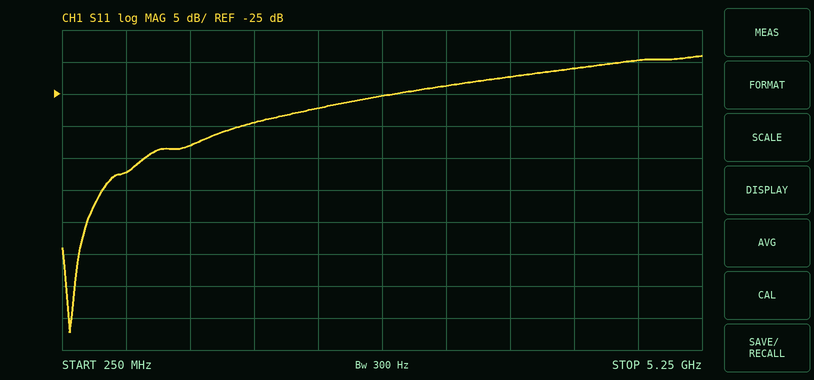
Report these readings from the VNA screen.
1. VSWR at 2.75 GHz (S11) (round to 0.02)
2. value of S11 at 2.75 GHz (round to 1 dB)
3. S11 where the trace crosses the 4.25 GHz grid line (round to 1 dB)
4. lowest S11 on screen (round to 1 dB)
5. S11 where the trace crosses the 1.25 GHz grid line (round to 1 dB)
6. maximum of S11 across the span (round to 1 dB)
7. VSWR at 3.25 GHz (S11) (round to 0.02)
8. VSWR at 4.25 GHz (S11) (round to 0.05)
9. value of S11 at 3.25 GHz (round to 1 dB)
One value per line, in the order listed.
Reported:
1.12
-25 dB
-21 dB
-62 dB
-33 dB
-19 dB
1.14
1.20
-24 dB
